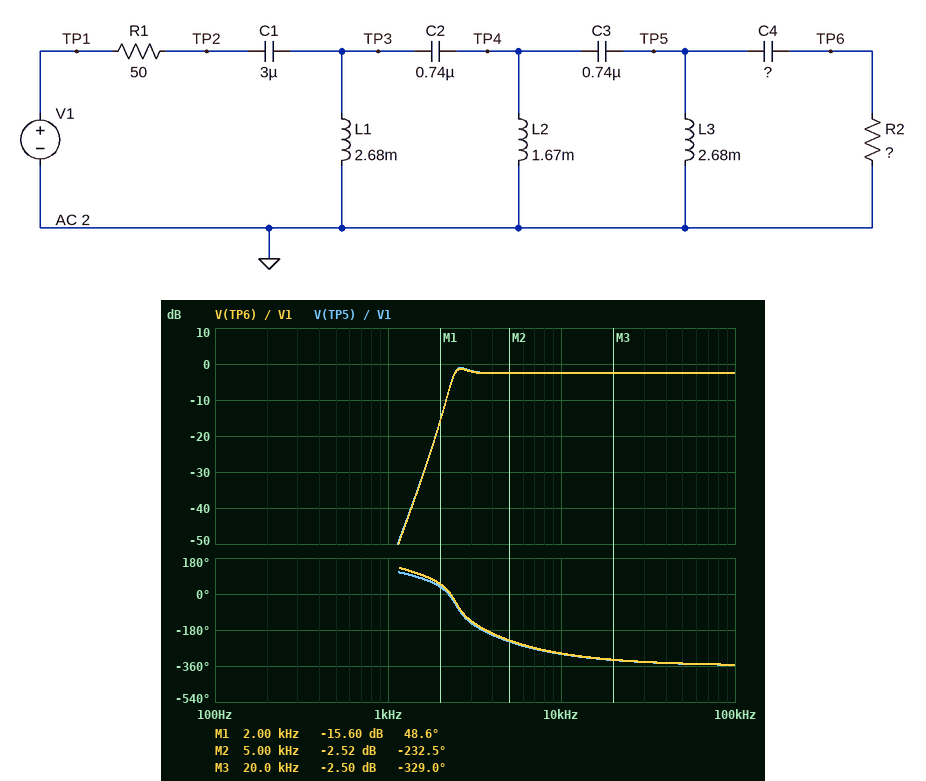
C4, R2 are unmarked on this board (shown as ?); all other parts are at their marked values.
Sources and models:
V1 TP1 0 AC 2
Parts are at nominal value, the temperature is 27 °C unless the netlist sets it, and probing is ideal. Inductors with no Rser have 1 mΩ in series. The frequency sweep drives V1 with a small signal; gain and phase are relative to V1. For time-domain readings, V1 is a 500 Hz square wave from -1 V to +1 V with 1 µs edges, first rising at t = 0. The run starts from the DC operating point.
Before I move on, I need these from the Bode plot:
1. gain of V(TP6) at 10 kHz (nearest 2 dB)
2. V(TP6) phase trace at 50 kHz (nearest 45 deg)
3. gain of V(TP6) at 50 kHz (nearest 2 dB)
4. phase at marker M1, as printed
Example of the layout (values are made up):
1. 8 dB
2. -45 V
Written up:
1. -2 dB
2. -360 deg
3. -2 dB
4. 48.6 deg
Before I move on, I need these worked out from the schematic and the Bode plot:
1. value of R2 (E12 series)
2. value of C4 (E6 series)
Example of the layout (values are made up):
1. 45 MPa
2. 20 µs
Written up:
1. 150 Ω
2. 2.2 µF
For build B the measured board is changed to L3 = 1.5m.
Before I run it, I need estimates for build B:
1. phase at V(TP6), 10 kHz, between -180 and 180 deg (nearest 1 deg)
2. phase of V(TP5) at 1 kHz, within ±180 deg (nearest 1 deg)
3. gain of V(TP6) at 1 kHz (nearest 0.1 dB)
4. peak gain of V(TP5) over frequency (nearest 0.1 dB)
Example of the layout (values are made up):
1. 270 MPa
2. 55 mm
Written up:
1. 72 deg
2. 122 deg
3. -63.2 dB
4. -2.5 dB
